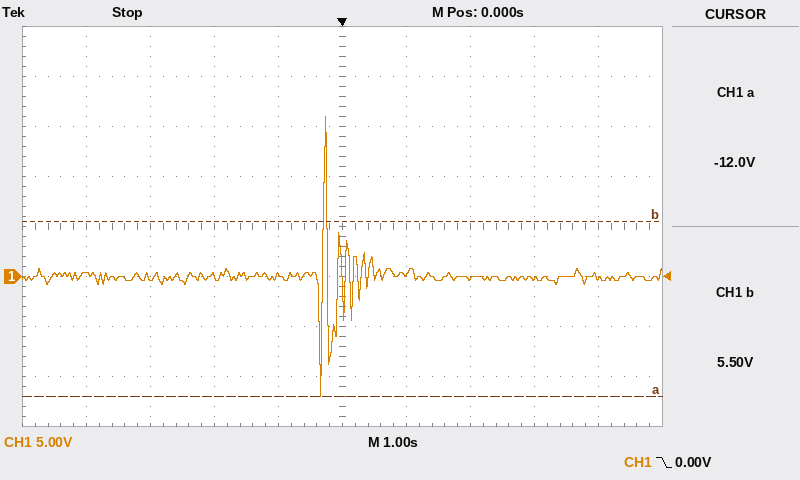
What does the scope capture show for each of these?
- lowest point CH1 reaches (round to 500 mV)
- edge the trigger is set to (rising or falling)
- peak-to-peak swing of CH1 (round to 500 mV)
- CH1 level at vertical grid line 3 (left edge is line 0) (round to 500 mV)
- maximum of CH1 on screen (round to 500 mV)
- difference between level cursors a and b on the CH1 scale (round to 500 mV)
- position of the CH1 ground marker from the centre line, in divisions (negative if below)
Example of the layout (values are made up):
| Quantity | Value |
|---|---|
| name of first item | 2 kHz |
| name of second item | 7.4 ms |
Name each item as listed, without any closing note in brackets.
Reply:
| Quantity | Value |
|---|---|
| lowest point CH1 reaches | -12.0 V |
| edge the trigger is set to | falling |
| peak-to-peak swing of CH1 | 28.0 V |
| CH1 level at vertical grid line 3 (left edge is line 0) | 0.0 V |
| maximum of CH1 on screen | 16.0 V |
| difference between level cursors a and b on the CH1 scale | 17.5 V |
| position of the CH1 ground marker from the centre line, in divisions | -1.0 div |
